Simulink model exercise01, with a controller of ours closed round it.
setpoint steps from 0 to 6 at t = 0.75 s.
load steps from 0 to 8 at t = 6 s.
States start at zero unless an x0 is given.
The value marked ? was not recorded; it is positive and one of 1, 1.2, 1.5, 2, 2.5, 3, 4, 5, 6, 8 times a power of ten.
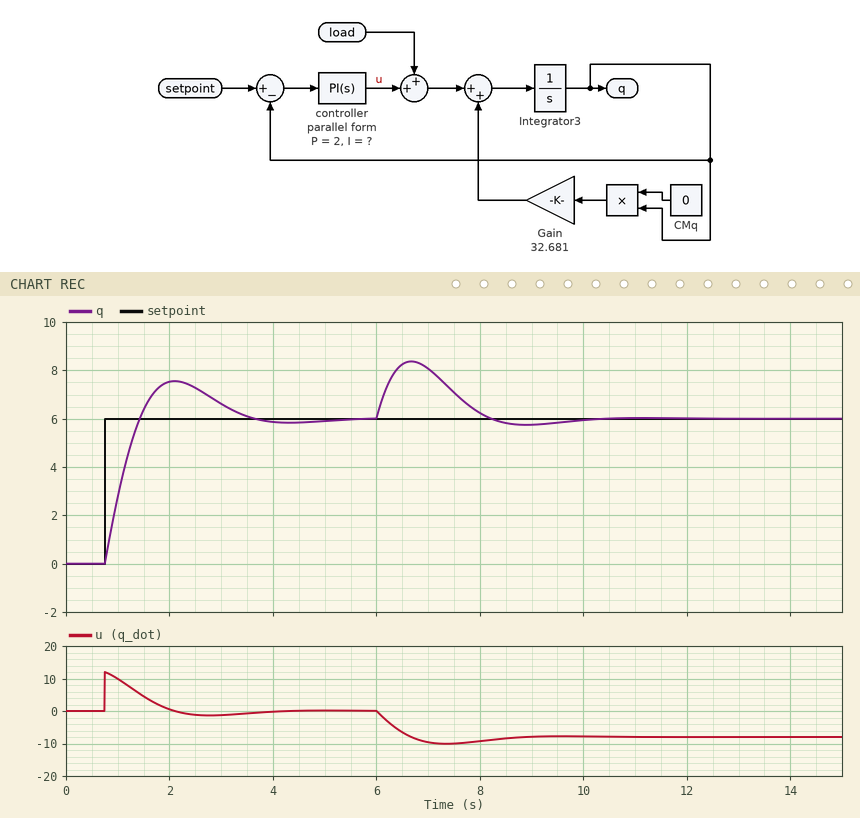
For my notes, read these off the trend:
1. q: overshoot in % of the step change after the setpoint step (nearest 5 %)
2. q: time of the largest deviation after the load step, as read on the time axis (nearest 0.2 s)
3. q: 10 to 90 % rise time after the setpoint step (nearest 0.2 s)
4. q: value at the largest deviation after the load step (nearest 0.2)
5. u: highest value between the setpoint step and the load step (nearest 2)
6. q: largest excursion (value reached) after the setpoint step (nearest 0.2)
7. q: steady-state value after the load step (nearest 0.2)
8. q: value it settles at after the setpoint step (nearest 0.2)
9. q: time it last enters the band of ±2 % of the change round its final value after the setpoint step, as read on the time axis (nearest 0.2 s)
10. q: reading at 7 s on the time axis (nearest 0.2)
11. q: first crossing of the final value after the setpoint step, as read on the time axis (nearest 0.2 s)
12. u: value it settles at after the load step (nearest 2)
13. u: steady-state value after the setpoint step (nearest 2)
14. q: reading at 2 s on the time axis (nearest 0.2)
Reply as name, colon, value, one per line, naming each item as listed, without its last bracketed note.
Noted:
q: overshoot in % of the step change after the setpoint step: 25 %
q: time of the largest deviation after the load step, as read on the time axis: 6.6 s
q: 10 to 90 % rise time after the setpoint step: 0.6 s
q: value at the largest deviation after the load step: 8.4
u: highest value between the setpoint step and the load step: 12
q: largest excursion (value reached) after the setpoint step: 7.6
q: steady-state value after the load step: 6.0
q: value it settles at after the setpoint step: 6.0
q: time it last enters the band of ±2 % of the change round its final value after the setpoint step, as read on the time axis: 4.8 s
q: reading at 7 s on the time axis: 8.0
q: first crossing of the final value after the setpoint step, as read on the time axis: 1.4 s
u: value it settles at after the load step: -8
u: steady-state value after the setpoint step: 0
q: reading at 2 s on the time axis: 7.6
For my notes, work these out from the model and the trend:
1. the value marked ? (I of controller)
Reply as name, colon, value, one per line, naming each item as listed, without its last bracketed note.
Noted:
the value marked ?: 3
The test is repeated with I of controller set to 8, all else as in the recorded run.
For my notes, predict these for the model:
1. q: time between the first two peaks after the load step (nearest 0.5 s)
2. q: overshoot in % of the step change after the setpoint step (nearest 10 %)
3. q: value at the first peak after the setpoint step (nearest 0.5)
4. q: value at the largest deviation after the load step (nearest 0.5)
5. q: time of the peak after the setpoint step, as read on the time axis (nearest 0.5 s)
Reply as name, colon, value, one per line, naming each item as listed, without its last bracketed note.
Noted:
q: time between the first two peaks after the load step: 2.5 s
q: overshoot in % of the step change after the setpoint step: 40 %
q: value at the first peak after the setpoint step: 8.5
q: value at the largest deviation after the load step: 8.0
q: time of the peak after the setpoint step, as read on the time axis: 1.5 s
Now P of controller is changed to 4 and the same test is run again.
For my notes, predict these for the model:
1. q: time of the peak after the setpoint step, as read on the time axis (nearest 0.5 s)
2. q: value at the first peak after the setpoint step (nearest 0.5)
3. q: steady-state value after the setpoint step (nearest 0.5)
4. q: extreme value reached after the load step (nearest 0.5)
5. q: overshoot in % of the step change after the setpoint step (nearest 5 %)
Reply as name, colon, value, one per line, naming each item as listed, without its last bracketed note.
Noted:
q: time of the peak after the setpoint step, as read on the time axis: 2.0 s
q: value at the first peak after the setpoint step: 6.5
q: steady-state value after the setpoint step: 6.0
q: extreme value reached after the load step: 7.5
q: overshoot in % of the step change after the setpoint step: 10 %
